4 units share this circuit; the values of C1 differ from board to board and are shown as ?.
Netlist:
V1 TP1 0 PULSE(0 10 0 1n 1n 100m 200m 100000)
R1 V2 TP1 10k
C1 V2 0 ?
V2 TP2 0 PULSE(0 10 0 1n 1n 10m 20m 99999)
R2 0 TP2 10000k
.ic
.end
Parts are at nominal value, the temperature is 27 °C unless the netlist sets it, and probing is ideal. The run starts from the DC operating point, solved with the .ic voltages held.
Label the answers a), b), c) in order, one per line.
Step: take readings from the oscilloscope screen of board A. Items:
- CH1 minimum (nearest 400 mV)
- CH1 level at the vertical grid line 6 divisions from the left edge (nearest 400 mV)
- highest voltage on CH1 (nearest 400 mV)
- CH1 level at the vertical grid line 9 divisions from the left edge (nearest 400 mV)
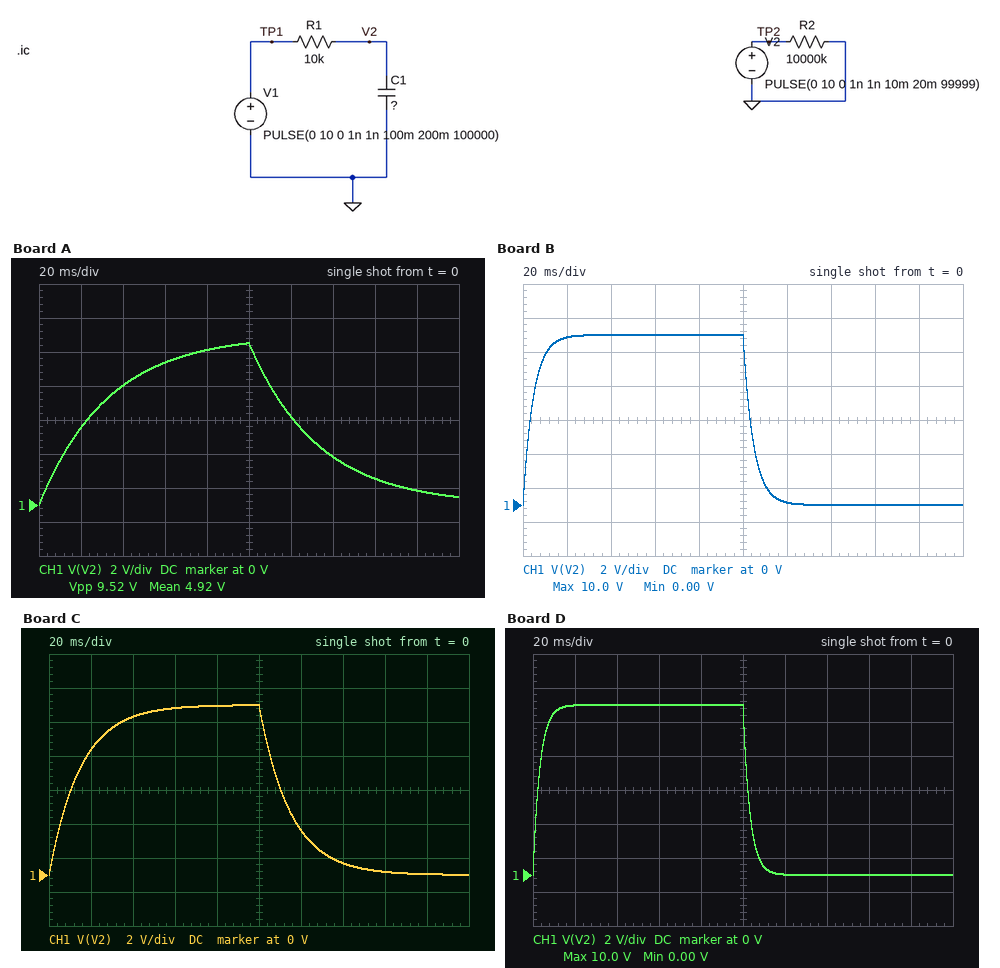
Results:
a) 0 V
b) 5.2 V
c) 9.6 V
d) 800 mV
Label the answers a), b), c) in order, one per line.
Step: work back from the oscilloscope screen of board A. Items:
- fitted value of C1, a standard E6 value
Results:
a) 3.3 µF
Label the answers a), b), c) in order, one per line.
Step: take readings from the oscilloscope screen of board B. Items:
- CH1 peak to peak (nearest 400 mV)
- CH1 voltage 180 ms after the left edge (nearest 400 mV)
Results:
a) 10.0 V
b) 0 V
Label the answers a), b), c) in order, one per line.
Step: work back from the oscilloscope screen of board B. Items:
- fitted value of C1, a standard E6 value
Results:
a) 470 nF
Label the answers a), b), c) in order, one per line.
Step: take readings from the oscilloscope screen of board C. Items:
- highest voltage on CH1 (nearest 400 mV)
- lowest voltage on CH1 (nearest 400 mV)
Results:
a) 10.0 V
b) 0 V
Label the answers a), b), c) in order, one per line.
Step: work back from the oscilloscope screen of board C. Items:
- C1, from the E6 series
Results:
a) 1.5 µF
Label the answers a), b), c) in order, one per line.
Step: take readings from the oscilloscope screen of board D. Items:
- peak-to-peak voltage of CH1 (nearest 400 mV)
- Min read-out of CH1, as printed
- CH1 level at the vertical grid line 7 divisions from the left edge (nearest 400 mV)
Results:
a) 10.0 V
b) 0.00 V
c) 0 V
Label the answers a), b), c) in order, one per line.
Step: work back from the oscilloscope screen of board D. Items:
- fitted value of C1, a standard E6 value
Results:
a) 330 nF
